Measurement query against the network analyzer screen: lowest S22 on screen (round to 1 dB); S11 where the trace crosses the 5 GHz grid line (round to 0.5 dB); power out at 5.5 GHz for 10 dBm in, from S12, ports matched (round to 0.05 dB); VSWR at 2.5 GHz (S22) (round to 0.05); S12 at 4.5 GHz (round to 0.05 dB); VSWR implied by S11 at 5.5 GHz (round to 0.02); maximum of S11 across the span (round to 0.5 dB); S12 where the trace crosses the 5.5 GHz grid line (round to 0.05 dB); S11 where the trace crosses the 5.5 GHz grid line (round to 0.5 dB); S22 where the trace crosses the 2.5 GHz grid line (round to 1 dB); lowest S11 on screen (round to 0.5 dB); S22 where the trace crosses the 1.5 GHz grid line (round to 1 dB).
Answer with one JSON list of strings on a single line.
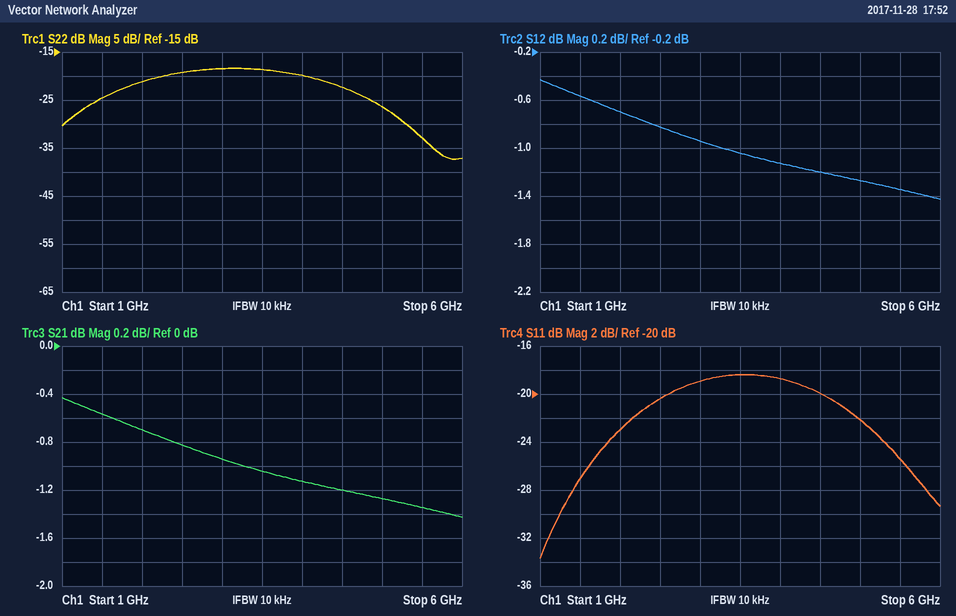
["-37 dB", "-22.0 dB", "8.65 dBm", "1.25", "-1.20 dB", "1.12", "-18.5 dB", "-1.35 dB", "-25.5 dB", "-19 dB", "-33.5 dB", "-25 dB"]
